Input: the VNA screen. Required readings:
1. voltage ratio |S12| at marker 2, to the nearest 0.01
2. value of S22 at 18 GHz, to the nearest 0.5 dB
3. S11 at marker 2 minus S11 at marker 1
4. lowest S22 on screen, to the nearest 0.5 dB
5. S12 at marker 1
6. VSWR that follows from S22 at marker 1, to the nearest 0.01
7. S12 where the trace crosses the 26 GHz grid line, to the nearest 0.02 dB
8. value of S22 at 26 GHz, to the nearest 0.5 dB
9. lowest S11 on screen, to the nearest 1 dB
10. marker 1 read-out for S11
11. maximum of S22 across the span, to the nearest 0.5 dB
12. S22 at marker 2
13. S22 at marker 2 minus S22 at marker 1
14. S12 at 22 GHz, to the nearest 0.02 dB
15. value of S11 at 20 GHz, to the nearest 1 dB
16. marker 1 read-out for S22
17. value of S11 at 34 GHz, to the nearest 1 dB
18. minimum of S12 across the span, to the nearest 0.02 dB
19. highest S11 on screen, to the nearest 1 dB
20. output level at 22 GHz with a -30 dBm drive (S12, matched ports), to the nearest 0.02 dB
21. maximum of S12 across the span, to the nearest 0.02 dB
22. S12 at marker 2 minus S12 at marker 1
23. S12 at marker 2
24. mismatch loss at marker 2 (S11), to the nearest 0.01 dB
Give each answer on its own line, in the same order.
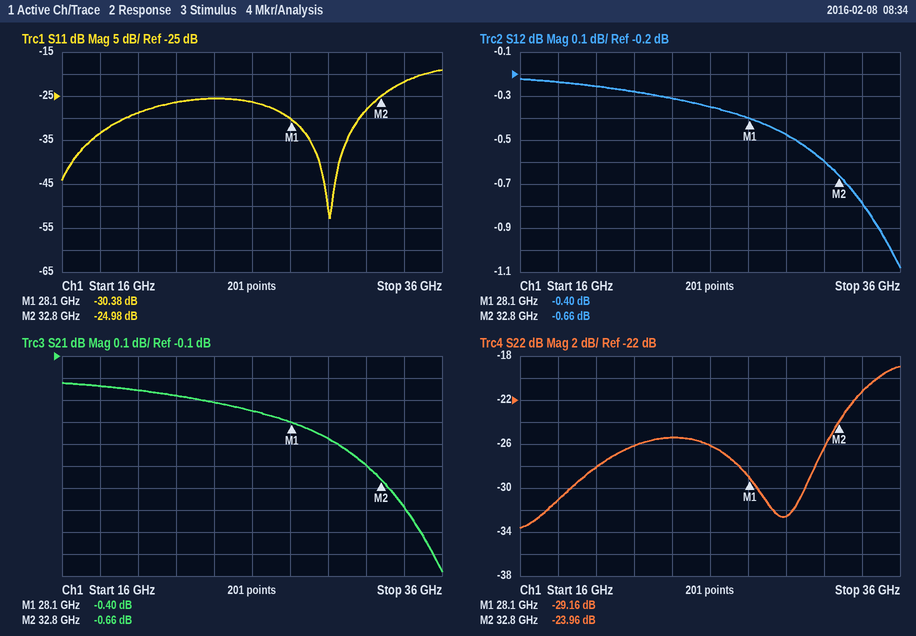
0.93
-31.0 dB
5.40 dB
-33.5 dB
-0.40 dB
1.07
-0.34 dB
-26.0 dB
-53 dB
-30.38 dB
-19.0 dB
-23.96 dB
5.20 dB
-0.28 dB
-29 dB
-29.16 dB
-22 dB
-1.08 dB
-19 dB
-30.28 dBm
-0.22 dB
-0.26 dB
-0.66 dB
0.01 dB
